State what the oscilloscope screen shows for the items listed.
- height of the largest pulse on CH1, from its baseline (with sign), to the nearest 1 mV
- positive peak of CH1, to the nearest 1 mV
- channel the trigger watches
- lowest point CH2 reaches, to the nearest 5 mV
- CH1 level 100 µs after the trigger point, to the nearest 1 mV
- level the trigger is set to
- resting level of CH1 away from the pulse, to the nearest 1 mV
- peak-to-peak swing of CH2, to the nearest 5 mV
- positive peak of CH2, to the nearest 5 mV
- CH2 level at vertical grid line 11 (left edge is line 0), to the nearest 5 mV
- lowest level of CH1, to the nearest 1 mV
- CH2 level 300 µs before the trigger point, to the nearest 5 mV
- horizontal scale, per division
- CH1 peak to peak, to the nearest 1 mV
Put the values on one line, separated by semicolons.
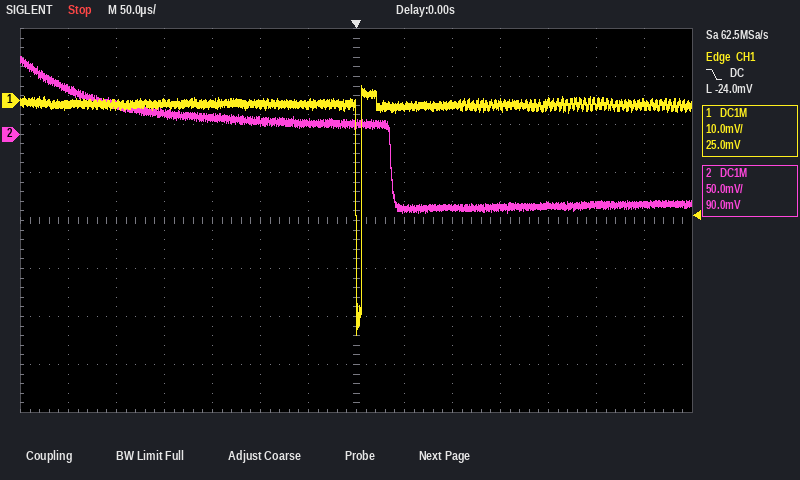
-48 mV; 3 mV; CH1; -85 mV; -1 mV; -24.0 mV; -1 mV; 165 mV; 80 mV; -75 mV; -49 mV; 45 mV; 50 µs; 52 mV
